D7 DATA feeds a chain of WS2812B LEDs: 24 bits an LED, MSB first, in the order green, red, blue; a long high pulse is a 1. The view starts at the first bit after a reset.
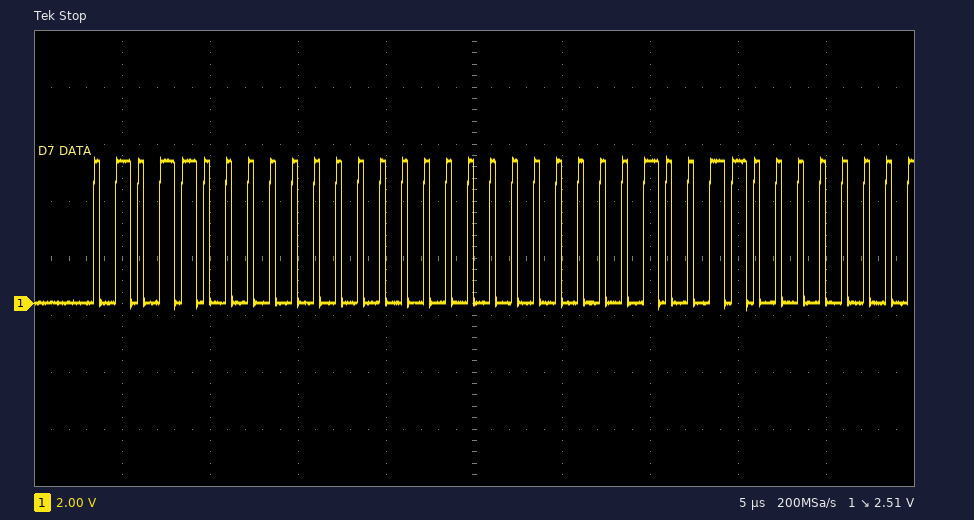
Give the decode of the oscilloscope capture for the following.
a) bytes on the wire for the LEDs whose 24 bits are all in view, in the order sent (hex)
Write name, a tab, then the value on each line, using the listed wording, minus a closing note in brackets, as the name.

bytes on the wire for the LEDs whose 24 bits are all in view, in the order sent	58 00 00
